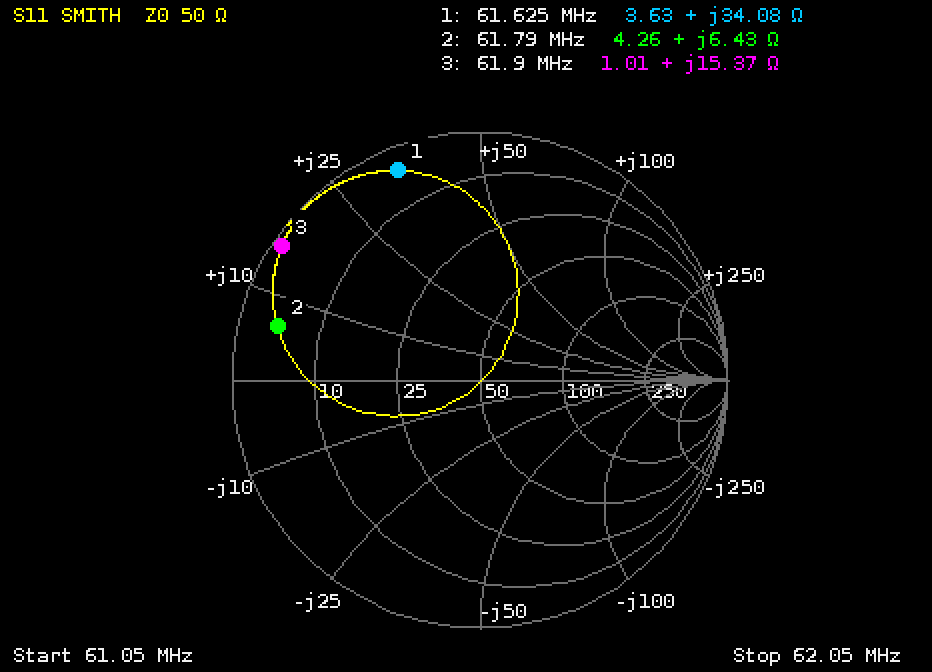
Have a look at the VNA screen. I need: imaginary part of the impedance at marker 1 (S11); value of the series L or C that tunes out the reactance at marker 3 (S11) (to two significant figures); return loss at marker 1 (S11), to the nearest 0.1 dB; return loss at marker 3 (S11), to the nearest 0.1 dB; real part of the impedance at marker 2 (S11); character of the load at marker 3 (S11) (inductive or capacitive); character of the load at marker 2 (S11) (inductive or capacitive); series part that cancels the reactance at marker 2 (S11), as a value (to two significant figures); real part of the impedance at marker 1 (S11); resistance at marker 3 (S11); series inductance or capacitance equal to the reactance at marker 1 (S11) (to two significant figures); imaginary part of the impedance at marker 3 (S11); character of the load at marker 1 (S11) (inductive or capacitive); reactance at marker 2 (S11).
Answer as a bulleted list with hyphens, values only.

- +34.08 Ω
- 170 pF
- 0.9 dB
- 0.3 dB
- 4.26 Ω
- inductive
- inductive
- 400 pF
- 3.63 Ω
- 1.01 Ω
- 88 nH
- +15.37 Ω
- inductive
- +6.43 Ω
